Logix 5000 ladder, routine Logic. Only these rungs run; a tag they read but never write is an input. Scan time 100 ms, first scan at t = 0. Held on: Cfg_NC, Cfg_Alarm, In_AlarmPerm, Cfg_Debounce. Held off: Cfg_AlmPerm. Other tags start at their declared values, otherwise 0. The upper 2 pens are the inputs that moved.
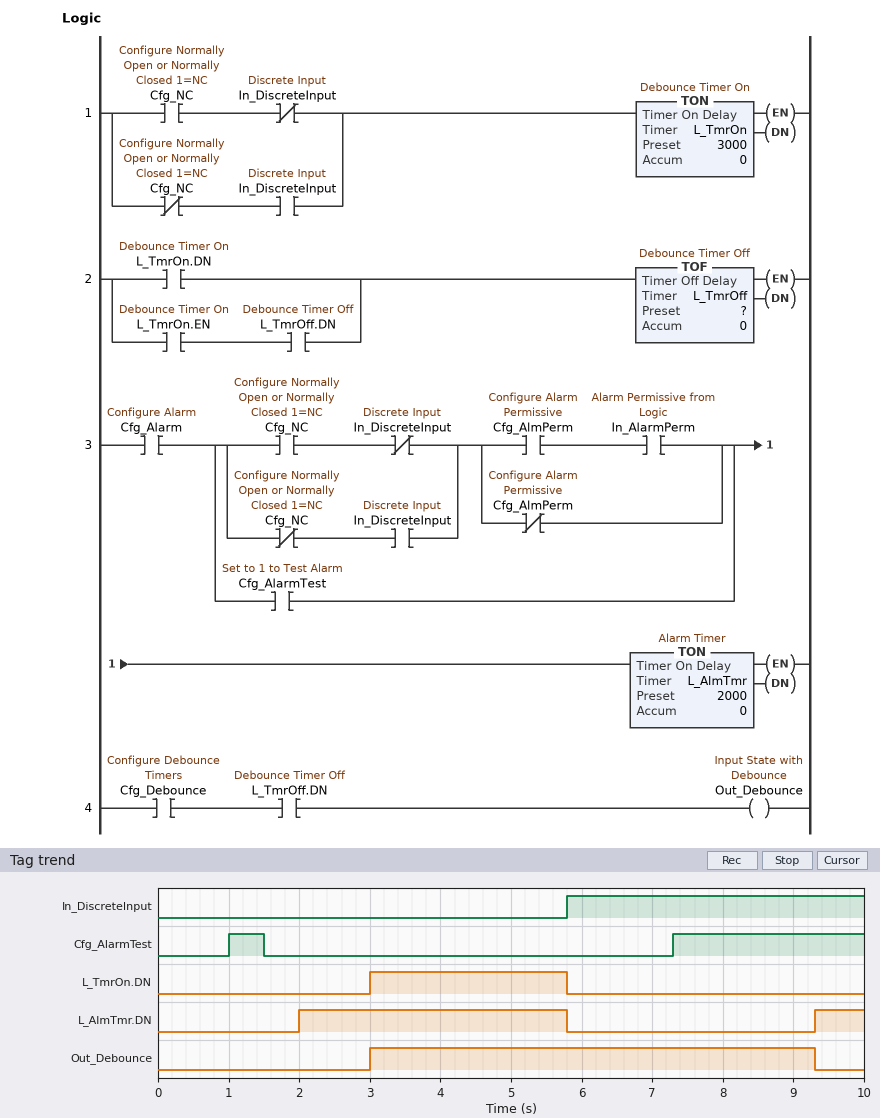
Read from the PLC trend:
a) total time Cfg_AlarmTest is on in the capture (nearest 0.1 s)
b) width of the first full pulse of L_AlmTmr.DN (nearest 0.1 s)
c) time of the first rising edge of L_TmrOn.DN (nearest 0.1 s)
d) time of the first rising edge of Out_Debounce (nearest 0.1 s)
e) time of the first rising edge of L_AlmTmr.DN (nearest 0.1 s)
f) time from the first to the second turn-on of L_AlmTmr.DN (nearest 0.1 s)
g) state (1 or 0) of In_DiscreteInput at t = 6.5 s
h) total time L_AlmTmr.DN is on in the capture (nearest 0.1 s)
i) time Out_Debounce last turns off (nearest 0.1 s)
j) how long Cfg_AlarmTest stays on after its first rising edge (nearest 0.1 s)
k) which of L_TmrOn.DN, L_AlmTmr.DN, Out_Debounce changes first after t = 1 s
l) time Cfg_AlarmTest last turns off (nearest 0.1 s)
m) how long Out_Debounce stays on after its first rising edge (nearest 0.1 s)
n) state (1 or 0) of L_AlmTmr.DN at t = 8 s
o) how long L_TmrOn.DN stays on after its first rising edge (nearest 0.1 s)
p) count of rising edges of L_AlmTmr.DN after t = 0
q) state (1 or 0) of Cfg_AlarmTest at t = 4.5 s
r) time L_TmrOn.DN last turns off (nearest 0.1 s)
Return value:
3.2 s
3.8 s
3.0 s
3.0 s
2.0 s
7.3 s
1
4.5 s
9.3 s
0.5 s
L_AlmTmr.DN
1.5 s
6.3 s
0
2.8 s
2
0
5.8 s
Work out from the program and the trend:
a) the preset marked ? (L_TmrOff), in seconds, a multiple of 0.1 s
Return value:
3.5 s
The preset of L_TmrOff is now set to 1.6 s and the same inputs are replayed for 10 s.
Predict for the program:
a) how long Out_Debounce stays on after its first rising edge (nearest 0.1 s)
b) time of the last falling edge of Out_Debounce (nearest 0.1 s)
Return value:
4.4 s
7.4 s
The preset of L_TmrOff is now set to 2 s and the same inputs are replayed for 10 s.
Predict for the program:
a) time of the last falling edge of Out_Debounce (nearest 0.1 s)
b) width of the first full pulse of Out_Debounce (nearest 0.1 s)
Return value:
7.8 s
4.8 s
